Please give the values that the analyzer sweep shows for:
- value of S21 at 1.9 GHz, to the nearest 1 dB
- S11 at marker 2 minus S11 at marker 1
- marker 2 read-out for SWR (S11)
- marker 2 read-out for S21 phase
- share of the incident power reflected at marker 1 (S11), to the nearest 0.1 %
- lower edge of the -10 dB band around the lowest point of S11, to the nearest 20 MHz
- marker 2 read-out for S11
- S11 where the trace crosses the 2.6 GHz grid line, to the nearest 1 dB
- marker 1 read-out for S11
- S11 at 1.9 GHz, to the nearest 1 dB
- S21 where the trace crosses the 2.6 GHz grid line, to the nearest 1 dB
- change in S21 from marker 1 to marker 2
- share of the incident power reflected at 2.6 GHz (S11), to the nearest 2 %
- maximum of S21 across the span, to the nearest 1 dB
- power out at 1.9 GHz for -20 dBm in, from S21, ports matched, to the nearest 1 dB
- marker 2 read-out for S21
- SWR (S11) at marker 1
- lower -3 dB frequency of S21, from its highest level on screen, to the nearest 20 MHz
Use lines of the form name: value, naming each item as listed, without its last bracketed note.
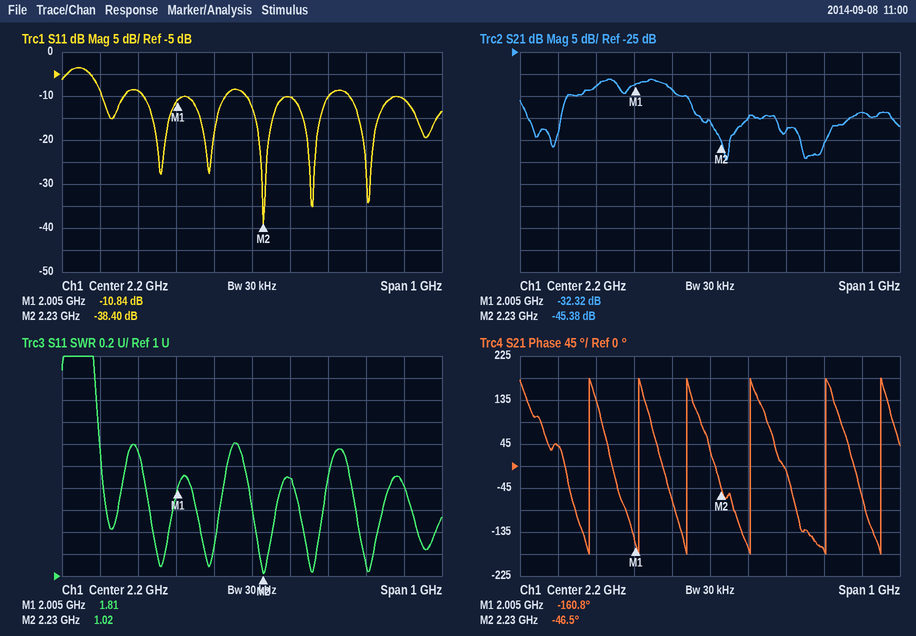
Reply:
value of S21 at 1.9 GHz, to the nearest 1 dB: -33 dB
S11 at marker 2 minus S11 at marker 1: -27.56 dB
marker 2 read-out for SWR: 1.02
marker 2 read-out for S21 phase: -46.5°
share of the incident power reflected at marker 1 (S11), to the nearest 0.1 %: 8.2 %
lower edge of the -10 dB band around the lowest point of S11, to the nearest 20 MHz: 2.18 GHz
marker 2 read-out for S11: -38.40 dB
S11 where the trace crosses the 2.6 GHz grid line, to the nearest 1 dB: -11 dB
marker 1 read-out for S11: -10.84 dB
S11 at 1.9 GHz, to the nearest 1 dB: -9 dB
S21 where the trace crosses the 2.6 GHz grid line, to the nearest 1 dB: -39 dB
change in S21 from marker 1 to marker 2: -13.06 dB
share of the incident power reflected at 2.6 GHz (S11), to the nearest 2 %: 8 %
maximum of S21 across the span, to the nearest 1 dB: -31 dB
power out at 1.9 GHz for -20 dBm in, from S21, ports matched, to the nearest 1 dB: -53 dBm
marker 2 read-out for S21: -45.38 dB
SWR (S11) at marker 1: 1.81
lower -3 dB frequency of S21, from its highest level on screen, to the nearest 20 MHz: 1.86 GHz
